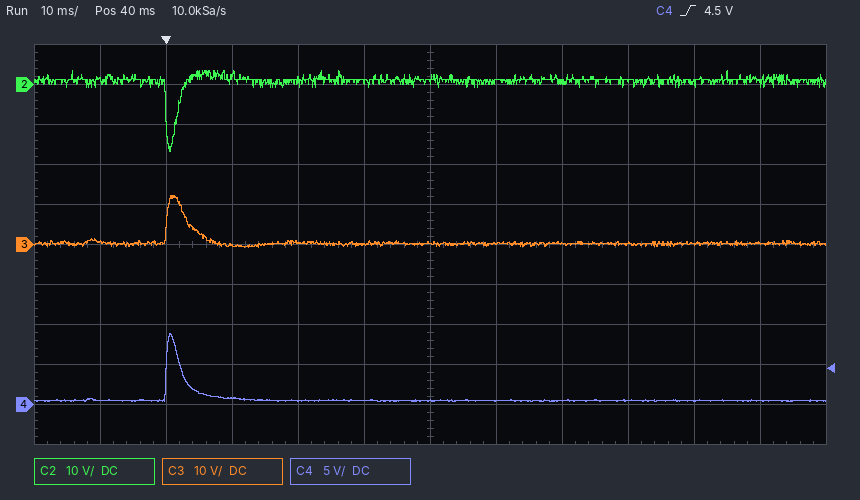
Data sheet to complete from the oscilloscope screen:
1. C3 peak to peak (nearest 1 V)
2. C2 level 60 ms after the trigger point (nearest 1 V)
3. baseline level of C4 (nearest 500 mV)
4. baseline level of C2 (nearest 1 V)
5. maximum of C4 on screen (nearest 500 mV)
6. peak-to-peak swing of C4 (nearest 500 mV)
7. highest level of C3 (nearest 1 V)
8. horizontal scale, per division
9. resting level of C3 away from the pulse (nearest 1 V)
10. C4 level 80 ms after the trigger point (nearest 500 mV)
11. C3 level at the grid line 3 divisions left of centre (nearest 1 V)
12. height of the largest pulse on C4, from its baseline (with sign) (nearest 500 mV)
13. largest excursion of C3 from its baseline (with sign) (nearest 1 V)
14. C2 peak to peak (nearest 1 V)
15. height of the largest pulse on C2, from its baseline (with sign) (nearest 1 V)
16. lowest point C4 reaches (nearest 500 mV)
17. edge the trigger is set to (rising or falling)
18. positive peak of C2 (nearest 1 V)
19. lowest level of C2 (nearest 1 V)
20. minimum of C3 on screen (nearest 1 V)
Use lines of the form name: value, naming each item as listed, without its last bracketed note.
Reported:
C3 peak to peak: 13 V
C2 level 60 ms after the trigger point: 1 V
baseline level of C4: 500 mV
baseline level of C2: 1 V
maximum of C4 on screen: 9.0 V
peak-to-peak swing of C4: 8.5 V
highest level of C3: 12 V
horizontal scale, per division: 10 ms
resting level of C3 away from the pulse: 0 V
C4 level 80 ms after the trigger point: 500 mV
C3 level at the grid line 3 divisions left of centre: 0 V
height of the largest pulse on C4, from its baseline (with sign): +8.5 V
largest excursion of C3 from its baseline (with sign): +12 V
C2 peak to peak: 20 V
height of the largest pulse on C2, from its baseline (with sign): -18 V
lowest point C4 reaches: 500 mV
edge the trigger is set to: rising
positive peak of C2: 3 V
lowest level of C2: -17 V
minimum of C3 on screen: -1 V
